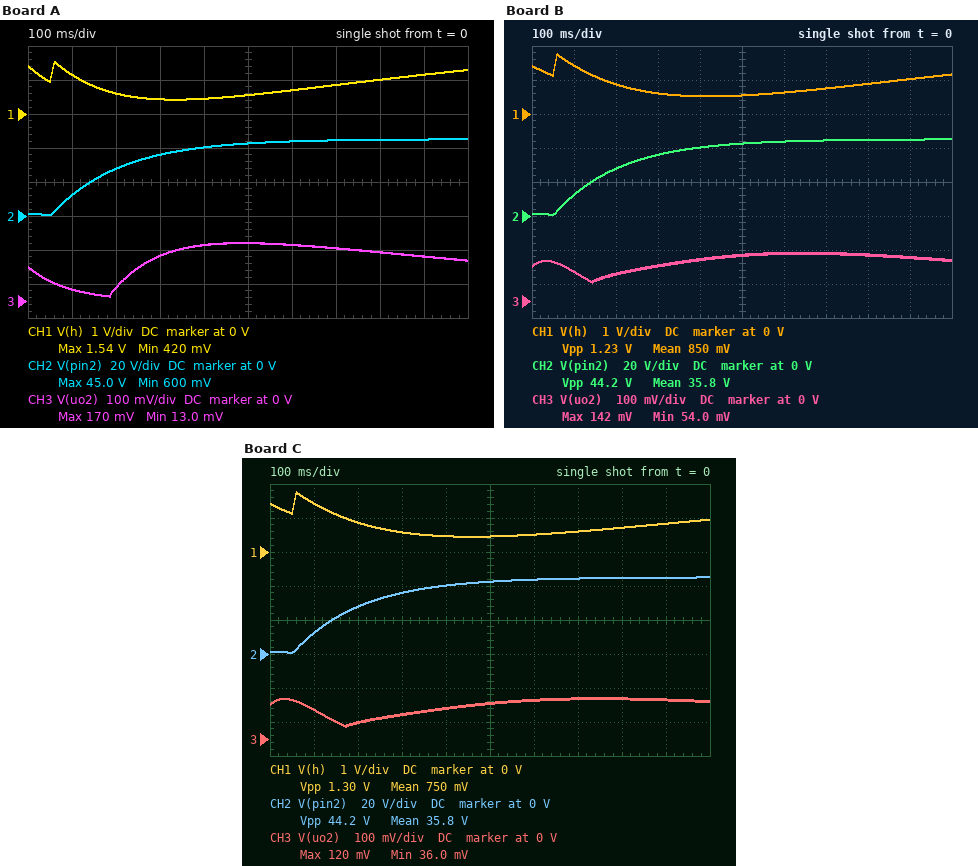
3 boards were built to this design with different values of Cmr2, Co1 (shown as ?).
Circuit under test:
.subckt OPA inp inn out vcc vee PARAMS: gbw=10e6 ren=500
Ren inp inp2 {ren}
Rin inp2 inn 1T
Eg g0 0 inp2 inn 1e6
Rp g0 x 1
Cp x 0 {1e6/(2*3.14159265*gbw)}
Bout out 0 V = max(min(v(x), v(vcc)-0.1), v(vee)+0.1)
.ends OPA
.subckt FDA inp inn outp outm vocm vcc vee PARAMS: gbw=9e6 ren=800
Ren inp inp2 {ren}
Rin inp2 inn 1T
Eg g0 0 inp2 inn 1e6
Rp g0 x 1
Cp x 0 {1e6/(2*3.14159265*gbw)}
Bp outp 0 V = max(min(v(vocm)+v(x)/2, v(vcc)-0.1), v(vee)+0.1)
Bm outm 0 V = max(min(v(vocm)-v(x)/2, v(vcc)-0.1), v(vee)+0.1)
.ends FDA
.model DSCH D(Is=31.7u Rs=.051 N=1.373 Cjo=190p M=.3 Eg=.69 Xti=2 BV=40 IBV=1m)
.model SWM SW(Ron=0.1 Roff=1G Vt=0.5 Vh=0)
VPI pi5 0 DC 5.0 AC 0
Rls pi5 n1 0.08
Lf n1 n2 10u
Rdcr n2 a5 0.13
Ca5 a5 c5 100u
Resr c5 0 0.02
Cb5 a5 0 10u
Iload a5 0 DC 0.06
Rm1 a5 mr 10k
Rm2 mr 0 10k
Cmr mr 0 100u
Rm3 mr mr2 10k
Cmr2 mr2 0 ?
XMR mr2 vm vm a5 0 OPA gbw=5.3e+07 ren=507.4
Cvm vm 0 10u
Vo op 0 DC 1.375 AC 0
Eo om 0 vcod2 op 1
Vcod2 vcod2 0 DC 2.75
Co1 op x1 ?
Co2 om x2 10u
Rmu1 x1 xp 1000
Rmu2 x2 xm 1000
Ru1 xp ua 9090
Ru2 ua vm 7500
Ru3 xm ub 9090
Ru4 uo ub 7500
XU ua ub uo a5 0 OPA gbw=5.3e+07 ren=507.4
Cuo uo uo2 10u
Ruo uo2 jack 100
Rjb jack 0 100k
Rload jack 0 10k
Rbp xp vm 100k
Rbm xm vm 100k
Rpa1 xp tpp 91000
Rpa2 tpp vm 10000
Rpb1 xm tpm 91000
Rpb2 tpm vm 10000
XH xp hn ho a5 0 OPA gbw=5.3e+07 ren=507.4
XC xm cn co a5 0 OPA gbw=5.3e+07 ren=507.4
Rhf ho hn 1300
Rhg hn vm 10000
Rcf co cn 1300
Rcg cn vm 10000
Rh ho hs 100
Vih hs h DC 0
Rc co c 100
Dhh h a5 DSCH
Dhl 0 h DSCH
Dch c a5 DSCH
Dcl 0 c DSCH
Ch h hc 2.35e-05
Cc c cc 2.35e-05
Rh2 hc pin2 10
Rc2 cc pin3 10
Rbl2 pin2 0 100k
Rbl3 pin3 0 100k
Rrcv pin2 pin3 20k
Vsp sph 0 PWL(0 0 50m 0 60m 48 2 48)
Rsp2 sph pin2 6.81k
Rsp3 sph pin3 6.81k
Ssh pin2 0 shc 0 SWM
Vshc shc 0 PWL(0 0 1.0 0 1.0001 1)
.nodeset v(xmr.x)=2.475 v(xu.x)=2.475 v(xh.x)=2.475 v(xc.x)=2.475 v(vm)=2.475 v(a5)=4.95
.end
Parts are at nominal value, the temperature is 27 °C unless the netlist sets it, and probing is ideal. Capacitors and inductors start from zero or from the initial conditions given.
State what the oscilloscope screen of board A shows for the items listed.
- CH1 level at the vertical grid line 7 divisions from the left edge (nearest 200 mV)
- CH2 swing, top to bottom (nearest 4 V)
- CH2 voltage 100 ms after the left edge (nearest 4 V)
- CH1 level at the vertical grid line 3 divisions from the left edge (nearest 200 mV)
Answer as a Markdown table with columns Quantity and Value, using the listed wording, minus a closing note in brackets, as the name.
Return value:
| Quantity | Value |
|---|---|
| CH1 level at the vertical grid line 7 divisions from the left edge | 800 mV |
| CH2 swing, top to bottom | 44 V |
| CH2 voltage 100 ms after the left edge | 12 V |
| CH1 level at the vertical grid line 3 divisions from the left edge | 400 mV |
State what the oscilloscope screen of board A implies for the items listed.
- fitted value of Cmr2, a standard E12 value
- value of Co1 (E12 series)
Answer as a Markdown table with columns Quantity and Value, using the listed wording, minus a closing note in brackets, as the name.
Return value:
| Quantity | Value |
|---|---|
| fitted value of Cmr2, a standard E12 value | 39 µF |
| value of Co1 | 8.2 µF |
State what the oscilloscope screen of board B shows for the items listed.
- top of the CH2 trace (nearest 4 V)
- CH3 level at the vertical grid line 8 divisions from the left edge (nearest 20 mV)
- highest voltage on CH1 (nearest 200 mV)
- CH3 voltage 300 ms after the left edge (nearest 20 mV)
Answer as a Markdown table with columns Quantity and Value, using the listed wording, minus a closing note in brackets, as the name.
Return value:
| Quantity | Value |
|---|---|
| top of the CH2 trace | 44 V |
| CH3 level at the vertical grid line 8 divisions from the left edge | 140 mV |
| highest voltage on CH1 | 1.8 V |
| CH3 voltage 300 ms after the left edge | 100 mV |
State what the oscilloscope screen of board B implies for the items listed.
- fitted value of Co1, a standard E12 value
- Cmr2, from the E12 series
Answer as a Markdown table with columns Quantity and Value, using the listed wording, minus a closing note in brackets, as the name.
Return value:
| Quantity | Value |
|---|---|
| fitted value of Co1, a standard E12 value | 15 µF |
| Cmr2, from the E12 series | 39 µF |
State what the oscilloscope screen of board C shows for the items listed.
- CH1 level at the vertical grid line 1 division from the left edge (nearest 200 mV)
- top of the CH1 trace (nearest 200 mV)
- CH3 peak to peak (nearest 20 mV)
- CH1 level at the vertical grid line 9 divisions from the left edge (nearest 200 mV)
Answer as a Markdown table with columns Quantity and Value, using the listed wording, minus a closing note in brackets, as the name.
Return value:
| Quantity | Value |
|---|---|
| CH1 level at the vertical grid line 1 division from the left edge | 1.4 V |
| top of the CH1 trace | 1.8 V |
| CH3 peak to peak | 80 mV |
| CH1 level at the vertical grid line 9 divisions from the left edge | 800 mV |
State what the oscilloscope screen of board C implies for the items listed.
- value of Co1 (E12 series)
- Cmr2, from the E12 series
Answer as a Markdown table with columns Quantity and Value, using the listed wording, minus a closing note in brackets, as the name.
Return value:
| Quantity | Value |
|---|---|
| value of Co1 | 15 µF |
| Cmr2, from the E12 series | 56 µF |
